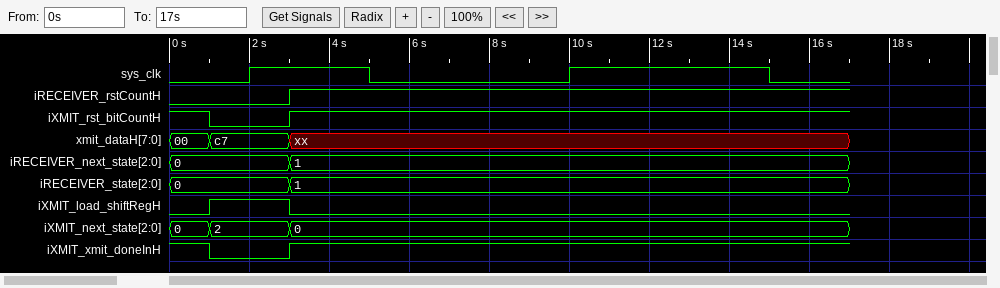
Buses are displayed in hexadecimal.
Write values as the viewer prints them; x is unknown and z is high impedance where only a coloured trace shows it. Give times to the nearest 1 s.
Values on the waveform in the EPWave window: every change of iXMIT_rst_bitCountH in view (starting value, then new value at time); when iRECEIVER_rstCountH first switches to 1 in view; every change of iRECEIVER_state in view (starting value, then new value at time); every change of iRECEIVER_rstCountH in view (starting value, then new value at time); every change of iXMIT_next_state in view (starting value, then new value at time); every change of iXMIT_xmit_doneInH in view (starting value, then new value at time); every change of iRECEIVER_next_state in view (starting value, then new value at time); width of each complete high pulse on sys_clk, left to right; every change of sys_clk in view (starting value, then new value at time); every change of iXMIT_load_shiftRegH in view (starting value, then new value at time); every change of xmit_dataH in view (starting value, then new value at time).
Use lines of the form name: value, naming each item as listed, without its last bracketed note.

every change of iXMIT_rst_bitCountH in view: 1, 0 at 1 s, 1 at 3 s
when iRECEIVER_rstCountH first switches to 1 in view: 3 s
every change of iRECEIVER_state in view: 0, 1 at 3 s
every change of iRECEIVER_rstCountH in view: 0, 1 at 3 s
every change of iXMIT_next_state in view: 0, 2 at 1 s, 0 at 3 s
every change of iXMIT_xmit_doneInH in view: 1, 0 at 1 s, 1 at 3 s
every change of iRECEIVER_next_state in view: 0, 1 at 3 s
width of each complete high pulse on sys_clk, left to right: 3 s, 5 s
every change of sys_clk in view: 0, 1 at 2 s, 0 at 5 s, 1 at 10 s, 0 at 15 s
every change of iXMIT_load_shiftRegH in view: 0, 1 at 1 s, 0 at 3 s
every change of xmit_dataH in view: 00, c7 at 1 s, xx at 3 s
